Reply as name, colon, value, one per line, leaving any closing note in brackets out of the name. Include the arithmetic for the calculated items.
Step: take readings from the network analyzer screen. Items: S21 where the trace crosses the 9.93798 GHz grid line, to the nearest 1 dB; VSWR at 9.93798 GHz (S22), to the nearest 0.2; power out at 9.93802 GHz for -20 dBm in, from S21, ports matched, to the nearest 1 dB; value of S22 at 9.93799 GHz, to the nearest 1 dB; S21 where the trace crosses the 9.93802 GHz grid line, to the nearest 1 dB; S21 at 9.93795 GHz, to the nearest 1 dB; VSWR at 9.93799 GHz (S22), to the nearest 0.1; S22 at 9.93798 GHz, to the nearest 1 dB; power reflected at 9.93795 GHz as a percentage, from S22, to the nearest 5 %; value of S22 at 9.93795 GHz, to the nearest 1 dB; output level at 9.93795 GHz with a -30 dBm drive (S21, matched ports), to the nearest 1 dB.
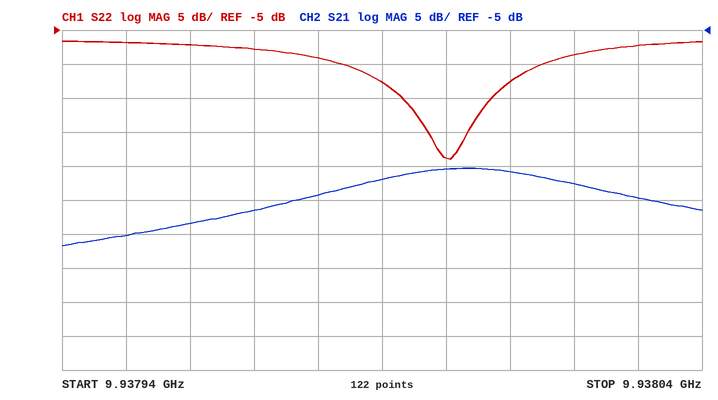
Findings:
S21 where the trace crosses the 9.93798 GHz grid line, to the nearest 1 dB: -29 dB
VSWR at 9.93798 GHz (S22), to the nearest 0.2: |Γ| = 10^(-9/20) = 0.3548; VSWR = (1 + 0.3548)/(1 − 0.3548) ≈ 2.10, so 2.0 to the nearest 0.2
power out at 9.93802 GHz for -20 dBm in, from S21, ports matched, to the nearest 1 dB: -20 dBm + (-28 dB) = -48 dBm
value of S22 at 9.93799 GHz, to the nearest 1 dB: -13 dB
S21 where the trace crosses the 9.93802 GHz grid line, to the nearest 1 dB: -28 dB
S21 at 9.93795 GHz, to the nearest 1 dB: -35 dB
VSWR at 9.93799 GHz (S22), to the nearest 0.1: |Γ| = 10^(-13/20) = 0.2239; VSWR = (1 + 0.2239)/(1 − 0.2239) ≈ 1.6
S22 at 9.93798 GHz, to the nearest 1 dB: -9 dB
power reflected at 9.93795 GHz as a percentage, from S22, to the nearest 5 %: 10^(-7/10) ≈ 20 %
value of S22 at 9.93795 GHz, to the nearest 1 dB: -7 dB
output level at 9.93795 GHz with a -30 dBm drive (S21, matched ports), to the nearest 1 dB: -30 dBm + (-35 dB) = -65 dBm
